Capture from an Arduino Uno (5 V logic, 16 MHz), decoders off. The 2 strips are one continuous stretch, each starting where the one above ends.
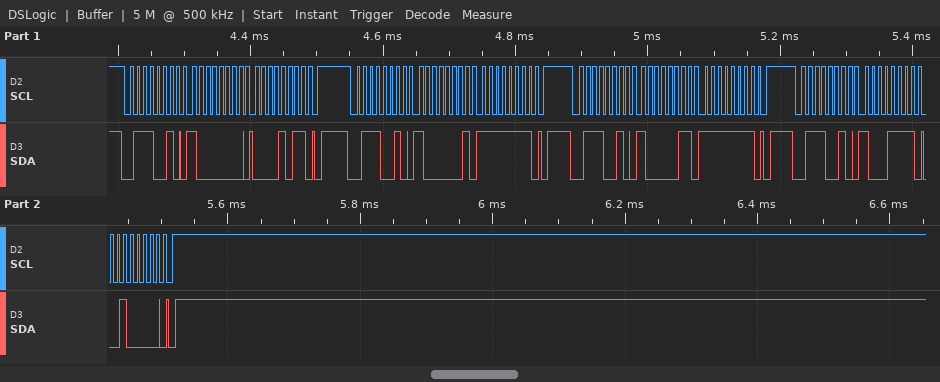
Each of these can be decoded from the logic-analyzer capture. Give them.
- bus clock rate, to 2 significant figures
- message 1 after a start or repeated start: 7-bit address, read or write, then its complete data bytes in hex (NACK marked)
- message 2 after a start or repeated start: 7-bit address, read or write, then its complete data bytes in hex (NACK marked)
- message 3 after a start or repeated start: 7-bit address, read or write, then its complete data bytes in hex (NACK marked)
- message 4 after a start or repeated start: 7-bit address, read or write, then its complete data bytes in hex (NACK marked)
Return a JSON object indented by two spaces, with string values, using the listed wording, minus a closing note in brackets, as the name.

{
  "bus clock rate, to 2 significant figures": "100 kHz",
  "message 1 after a start or repeated start: 7-bit address, read or write, then its complete data bytes in hex": "0x39 write: 80 0B",
  "message 2 after a start or repeated start: 7-bit address, read or write, then its complete data bytes in hex": "0x39 write: 81 FF",
  "message 3 after a start or repeated start: 7-bit address, read or write, then its complete data bytes in hex": "0x39 write: 83 FF",
  "message 4 after a start or repeated start: 7-bit address, read or write, then its complete data bytes in hex": "0x39 write: 8F 20"
}
